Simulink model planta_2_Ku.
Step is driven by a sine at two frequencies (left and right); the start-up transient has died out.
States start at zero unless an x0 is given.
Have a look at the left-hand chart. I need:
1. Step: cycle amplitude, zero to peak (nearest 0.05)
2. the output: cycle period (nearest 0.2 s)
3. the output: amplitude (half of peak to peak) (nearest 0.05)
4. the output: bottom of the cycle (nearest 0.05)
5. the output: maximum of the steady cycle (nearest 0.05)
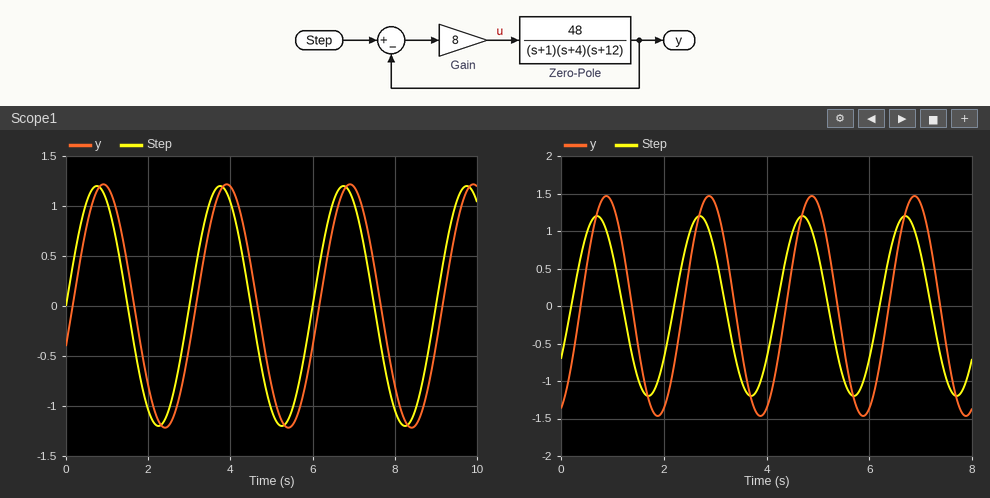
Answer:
1.20
3.0 s
1.20
-1.20
1.20
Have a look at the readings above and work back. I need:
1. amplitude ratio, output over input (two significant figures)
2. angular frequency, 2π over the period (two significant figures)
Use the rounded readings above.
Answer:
1.0
2.1 rad/s
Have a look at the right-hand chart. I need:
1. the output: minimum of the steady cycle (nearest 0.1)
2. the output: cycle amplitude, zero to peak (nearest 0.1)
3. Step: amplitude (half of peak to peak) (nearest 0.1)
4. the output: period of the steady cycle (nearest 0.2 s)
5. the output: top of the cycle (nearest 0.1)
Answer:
-1.5
1.5
1.2
2.0 s
1.5
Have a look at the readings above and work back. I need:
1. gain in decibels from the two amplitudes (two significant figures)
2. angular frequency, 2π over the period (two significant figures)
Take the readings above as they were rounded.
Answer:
1.9 dB
3.1 rad/s
